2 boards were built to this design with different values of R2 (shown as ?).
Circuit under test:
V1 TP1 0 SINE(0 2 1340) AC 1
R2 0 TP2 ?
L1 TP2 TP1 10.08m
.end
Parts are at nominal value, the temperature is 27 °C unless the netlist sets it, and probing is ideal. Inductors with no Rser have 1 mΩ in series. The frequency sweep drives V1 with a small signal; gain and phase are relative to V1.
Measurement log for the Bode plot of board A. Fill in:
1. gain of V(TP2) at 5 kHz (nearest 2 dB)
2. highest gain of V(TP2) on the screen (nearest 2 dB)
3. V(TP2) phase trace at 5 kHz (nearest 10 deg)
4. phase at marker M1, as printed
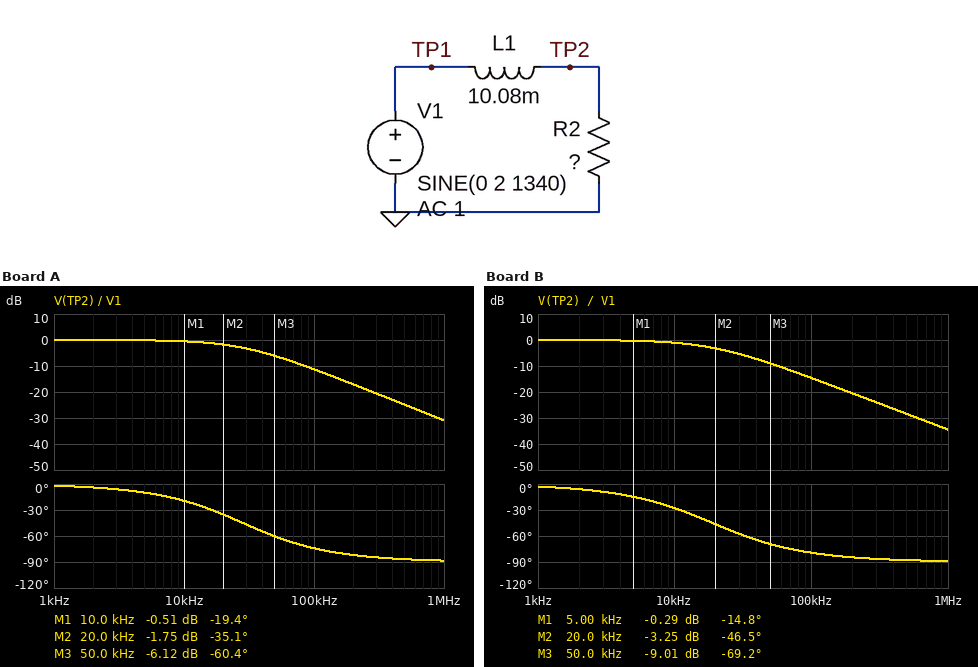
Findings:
0 dB
0 dB
-10 deg
-19.4 deg
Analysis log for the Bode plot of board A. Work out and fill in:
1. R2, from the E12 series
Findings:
1.8 kΩ
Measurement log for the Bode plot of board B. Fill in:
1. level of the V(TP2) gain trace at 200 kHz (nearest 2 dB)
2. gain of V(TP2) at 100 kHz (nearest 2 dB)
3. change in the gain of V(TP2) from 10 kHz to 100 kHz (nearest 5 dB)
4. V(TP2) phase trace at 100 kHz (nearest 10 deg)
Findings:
-20 dB
-14 dB
-15 dB
-80 deg
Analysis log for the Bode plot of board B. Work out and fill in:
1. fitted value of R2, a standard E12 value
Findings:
1.2 kΩ
